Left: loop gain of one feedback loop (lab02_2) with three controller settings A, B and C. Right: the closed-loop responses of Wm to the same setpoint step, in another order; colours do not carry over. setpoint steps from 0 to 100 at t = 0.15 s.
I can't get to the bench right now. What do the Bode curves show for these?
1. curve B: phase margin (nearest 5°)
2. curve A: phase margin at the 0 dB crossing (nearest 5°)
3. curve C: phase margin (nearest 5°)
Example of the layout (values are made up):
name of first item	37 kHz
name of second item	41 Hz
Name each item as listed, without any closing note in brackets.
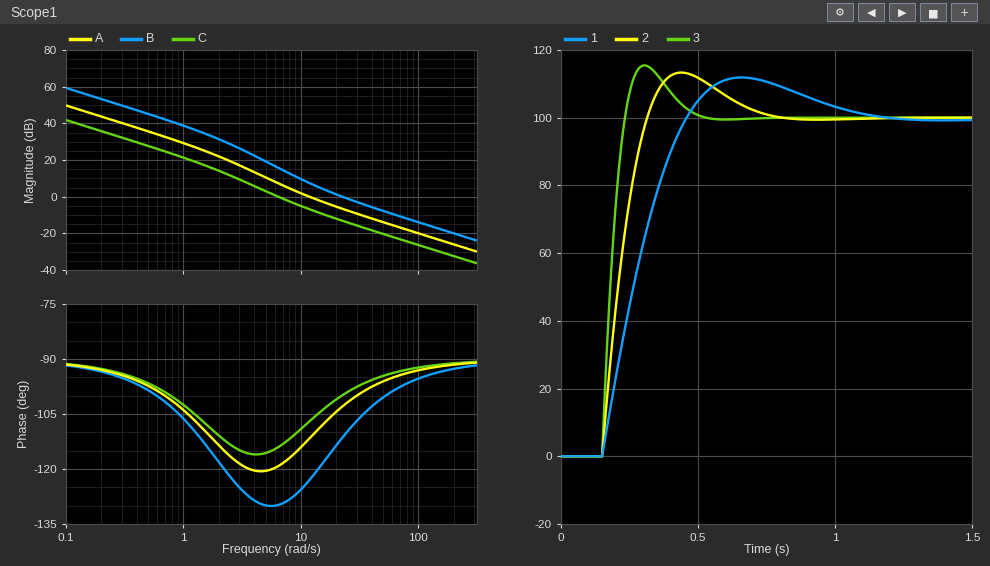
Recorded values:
curve B: phase margin	70°
curve A: phase margin at the 0 dB crossing	70°
curve C: phase margin	65°
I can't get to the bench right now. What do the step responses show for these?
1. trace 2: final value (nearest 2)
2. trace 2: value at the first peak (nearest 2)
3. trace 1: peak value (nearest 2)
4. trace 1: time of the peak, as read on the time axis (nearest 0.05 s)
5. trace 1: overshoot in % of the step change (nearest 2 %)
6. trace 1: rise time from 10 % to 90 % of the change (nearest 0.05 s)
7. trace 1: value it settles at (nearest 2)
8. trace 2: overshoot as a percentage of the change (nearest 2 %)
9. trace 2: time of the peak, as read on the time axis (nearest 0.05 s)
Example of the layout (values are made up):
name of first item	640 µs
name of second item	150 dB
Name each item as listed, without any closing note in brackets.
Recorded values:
trace 2: final value	100
trace 2: value at the first peak	114
trace 1: peak value	112
trace 1: time of the peak, as read on the time axis	0.65 s
trace 1: overshoot in % of the step change	12 %
trace 1: rise time from 10 % to 90 % of the change	0.25 s
trace 1: value it settles at	100
trace 2: overshoot as a percentage of the change	14 %
trace 2: time of the peak, as read on the time axis	0.45 s
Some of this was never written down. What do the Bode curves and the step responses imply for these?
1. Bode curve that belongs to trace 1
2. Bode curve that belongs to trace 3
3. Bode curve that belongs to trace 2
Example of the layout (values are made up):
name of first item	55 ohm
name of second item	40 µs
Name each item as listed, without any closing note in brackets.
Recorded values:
Bode curve that belongs to trace 1	C
Bode curve that belongs to trace 3	B
Bode curve that belongs to trace 2	A
